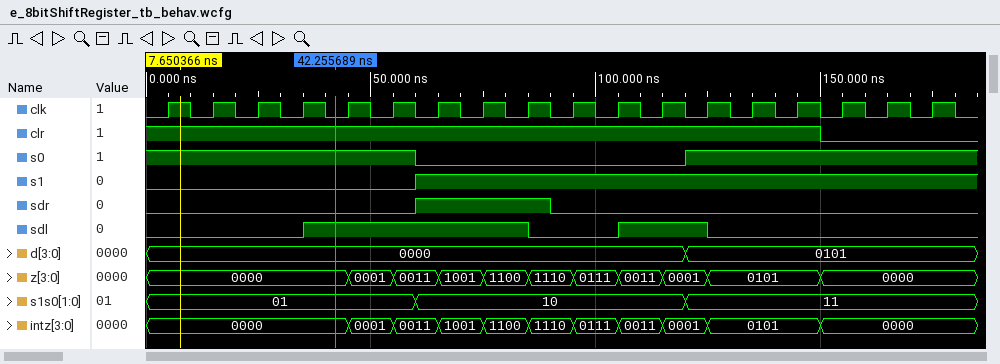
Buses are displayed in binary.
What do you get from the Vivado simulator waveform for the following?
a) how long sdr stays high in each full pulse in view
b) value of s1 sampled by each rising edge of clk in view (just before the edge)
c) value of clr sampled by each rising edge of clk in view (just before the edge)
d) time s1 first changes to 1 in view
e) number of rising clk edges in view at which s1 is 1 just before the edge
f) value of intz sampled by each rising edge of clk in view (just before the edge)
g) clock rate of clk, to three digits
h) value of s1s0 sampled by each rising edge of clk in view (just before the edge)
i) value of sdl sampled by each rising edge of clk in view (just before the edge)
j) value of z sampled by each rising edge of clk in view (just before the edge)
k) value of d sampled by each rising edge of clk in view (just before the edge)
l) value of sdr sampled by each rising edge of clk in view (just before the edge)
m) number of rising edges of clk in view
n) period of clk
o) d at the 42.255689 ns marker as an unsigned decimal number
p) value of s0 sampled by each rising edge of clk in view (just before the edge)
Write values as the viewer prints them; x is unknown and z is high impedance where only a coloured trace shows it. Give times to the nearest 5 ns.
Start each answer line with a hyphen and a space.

- 30 ns
- 0 0 0 0 0 0 1 1 1 1 1 1 1 1 1 1 1 1
- 1 1 1 1 1 1 1 1 1 1 1 1 1 1 1 0 0 0
- 60 ns
- 12
- 0000, 0000, 0000, 0000, 0000, 0001, 0011, 1001, 1100, 1110, 0111, 0011, 0001, 0101, 0101, 0000, 0000, 0000
- 100 MHz
- 01, 01, 01, 01, 01, 01, 10, 10, 10, 10, 10, 10, 11, 11, 11, 11, 11, 11
- 0 0 0 0 1 1 1 1 1 0 0 1 1 0 0 0 0 0
- 0000, 0000, 0000, 0000, 0000, 0001, 0011, 1001, 1100, 1110, 0111, 0011, 0001, 0101, 0101, 0000, 0000, 0000
- 0000, 0000, 0000, 0000, 0000, 0000, 0000, 0000, 0000, 0000, 0000, 0000, 0101, 0101, 0101, 0101, 0101, 0101
- 0 0 0 0 0 0 1 1 1 0 0 0 0 0 0 0 0 0
- 18
- 10 ns
- 0
- 1 1 1 1 1 1 0 0 0 0 0 0 1 1 1 1 1 1
